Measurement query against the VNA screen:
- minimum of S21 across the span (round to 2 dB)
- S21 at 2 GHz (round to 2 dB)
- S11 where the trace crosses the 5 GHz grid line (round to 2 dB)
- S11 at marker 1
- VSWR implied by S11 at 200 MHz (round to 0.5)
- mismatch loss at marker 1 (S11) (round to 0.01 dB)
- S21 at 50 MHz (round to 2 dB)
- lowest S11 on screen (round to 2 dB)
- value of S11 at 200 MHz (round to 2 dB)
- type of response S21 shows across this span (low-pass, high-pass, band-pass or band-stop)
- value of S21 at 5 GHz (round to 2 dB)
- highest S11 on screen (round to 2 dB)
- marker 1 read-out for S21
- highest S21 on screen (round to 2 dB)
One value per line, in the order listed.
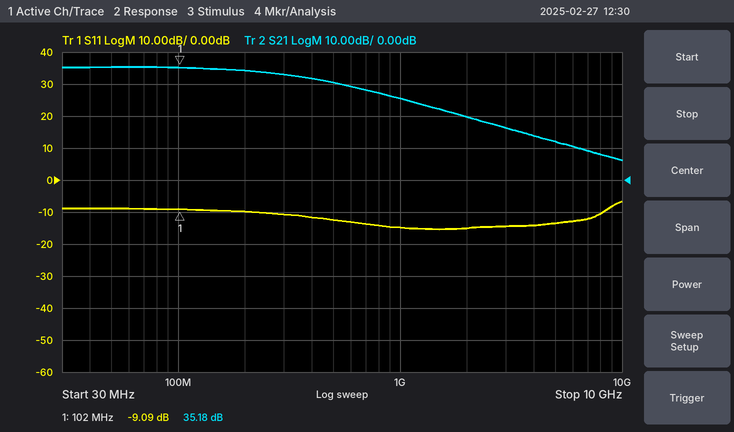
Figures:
6 dB
20 dB
-14 dB
-9.09 dB
2.0
0.57 dB
36 dB
-16 dB
-10 dB
low-pass
12 dB
-6 dB
35.18 dB
36 dB
